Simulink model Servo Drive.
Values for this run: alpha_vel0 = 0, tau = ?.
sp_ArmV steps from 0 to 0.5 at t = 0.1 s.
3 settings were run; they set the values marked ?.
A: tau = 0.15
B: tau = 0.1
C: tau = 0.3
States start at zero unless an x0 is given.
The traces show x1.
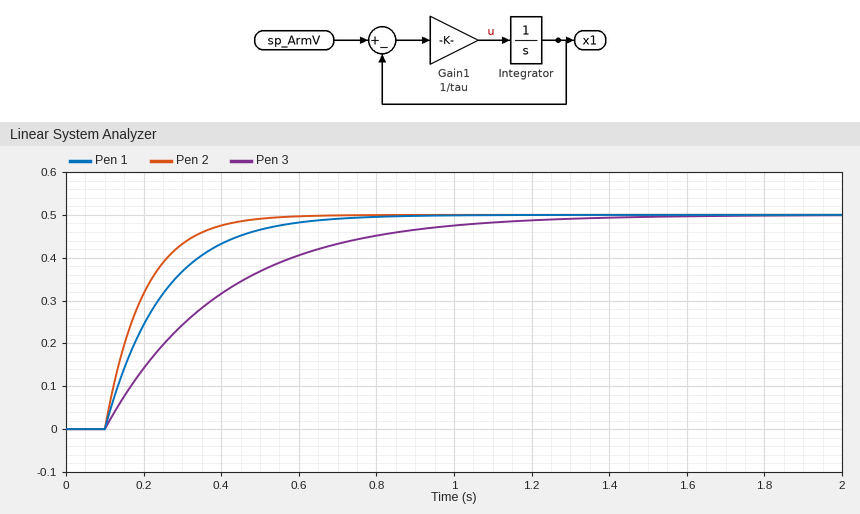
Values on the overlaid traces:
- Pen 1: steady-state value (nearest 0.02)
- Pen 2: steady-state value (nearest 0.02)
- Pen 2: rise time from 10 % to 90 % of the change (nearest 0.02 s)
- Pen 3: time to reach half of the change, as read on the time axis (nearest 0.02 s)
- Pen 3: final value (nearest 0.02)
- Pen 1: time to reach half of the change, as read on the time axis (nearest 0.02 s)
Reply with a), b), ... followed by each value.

a) 0.50
b) 0.50
c) 0.22 s
d) 0.30 s
e) 0.50
f) 0.20 s
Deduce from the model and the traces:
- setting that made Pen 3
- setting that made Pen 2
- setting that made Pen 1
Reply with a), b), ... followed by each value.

a) C
b) B
c) A
